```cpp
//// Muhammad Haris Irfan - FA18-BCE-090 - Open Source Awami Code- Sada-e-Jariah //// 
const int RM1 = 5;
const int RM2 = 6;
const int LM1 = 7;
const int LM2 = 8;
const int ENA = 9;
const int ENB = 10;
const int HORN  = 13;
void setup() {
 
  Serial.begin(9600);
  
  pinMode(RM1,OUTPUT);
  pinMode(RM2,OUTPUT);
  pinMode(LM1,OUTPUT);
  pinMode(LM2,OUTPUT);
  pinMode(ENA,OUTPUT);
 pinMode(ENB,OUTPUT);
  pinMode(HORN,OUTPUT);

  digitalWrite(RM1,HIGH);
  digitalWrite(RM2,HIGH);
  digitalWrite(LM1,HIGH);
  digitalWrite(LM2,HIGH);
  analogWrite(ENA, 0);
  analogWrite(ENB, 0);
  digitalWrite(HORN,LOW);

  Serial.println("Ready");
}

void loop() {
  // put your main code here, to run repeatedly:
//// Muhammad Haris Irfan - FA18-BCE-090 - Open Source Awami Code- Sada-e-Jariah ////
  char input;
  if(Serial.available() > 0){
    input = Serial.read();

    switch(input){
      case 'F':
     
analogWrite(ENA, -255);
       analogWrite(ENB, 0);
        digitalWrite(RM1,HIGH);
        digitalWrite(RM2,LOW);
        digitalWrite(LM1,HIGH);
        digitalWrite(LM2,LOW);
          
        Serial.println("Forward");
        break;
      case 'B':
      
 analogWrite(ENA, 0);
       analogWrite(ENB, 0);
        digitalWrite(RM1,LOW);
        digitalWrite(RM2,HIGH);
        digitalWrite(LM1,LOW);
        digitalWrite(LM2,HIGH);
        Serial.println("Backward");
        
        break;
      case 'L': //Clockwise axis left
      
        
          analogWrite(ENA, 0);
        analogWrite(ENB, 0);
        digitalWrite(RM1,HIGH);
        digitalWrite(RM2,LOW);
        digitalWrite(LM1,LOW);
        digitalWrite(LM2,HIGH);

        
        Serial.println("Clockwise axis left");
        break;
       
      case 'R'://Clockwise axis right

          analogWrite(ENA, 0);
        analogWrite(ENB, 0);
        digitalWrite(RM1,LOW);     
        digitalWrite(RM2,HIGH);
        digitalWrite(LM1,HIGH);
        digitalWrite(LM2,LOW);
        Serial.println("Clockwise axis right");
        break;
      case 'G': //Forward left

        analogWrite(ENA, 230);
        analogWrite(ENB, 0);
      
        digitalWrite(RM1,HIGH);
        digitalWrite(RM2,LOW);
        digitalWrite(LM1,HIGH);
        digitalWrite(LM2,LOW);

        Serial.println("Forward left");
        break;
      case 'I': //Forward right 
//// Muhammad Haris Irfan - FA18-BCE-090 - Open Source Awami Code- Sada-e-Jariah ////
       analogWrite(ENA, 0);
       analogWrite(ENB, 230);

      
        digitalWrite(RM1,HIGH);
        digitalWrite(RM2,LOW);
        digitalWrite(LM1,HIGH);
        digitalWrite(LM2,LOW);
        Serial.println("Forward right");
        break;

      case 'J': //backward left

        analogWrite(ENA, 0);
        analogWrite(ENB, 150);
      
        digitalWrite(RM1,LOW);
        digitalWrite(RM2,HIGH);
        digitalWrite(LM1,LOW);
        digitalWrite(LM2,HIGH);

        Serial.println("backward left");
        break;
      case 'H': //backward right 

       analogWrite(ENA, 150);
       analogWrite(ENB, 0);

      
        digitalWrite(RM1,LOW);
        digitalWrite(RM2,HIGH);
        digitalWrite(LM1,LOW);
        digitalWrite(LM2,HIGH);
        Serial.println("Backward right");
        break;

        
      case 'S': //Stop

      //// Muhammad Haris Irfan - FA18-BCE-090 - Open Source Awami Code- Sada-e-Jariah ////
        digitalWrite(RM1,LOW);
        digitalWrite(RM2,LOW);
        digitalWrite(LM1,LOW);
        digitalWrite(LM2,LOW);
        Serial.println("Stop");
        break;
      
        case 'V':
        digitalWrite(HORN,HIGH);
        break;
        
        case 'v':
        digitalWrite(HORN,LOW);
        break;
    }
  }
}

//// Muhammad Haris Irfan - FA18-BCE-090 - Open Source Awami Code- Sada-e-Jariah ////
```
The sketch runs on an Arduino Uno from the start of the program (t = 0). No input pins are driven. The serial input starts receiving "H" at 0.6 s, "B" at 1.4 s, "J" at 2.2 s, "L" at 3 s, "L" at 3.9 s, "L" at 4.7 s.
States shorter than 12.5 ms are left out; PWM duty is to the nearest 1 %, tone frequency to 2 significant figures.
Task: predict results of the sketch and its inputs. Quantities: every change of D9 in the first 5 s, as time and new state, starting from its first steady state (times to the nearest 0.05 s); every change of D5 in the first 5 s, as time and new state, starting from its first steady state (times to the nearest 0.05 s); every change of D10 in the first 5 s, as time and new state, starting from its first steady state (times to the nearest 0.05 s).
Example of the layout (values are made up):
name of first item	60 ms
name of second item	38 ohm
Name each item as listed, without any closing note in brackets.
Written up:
every change of D9 in the first 5 s, as time and new state, starting from its first steady state	0 s low; 0.6 s PWM 59 %; 1.4 s low
every change of D5 in the first 5 s, as time and new state, starting from its first steady state	0 s high; 0.6 s low; 3 s high
every change of D10 in the first 5 s, as time and new state, starting from its first steady state	0 s low; 2.2 s PWM 59 %; 3 s low
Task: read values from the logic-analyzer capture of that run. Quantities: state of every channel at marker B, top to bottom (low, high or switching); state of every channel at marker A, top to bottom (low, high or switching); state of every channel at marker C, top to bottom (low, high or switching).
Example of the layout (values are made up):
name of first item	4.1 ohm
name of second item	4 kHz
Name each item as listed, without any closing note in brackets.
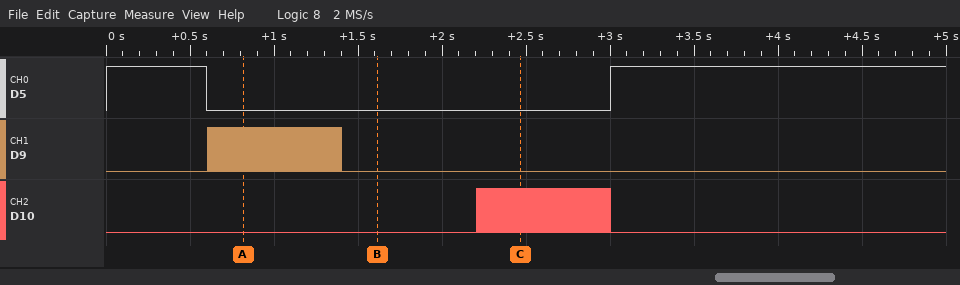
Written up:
state of every channel at marker B, top to bottom	D5 low, D9 low, D10 low
state of every channel at marker A, top to bottom	D5 low, D9 switching, D10 low
state of every channel at marker C, top to bottom	D5 low, D9 low, D10 switching
